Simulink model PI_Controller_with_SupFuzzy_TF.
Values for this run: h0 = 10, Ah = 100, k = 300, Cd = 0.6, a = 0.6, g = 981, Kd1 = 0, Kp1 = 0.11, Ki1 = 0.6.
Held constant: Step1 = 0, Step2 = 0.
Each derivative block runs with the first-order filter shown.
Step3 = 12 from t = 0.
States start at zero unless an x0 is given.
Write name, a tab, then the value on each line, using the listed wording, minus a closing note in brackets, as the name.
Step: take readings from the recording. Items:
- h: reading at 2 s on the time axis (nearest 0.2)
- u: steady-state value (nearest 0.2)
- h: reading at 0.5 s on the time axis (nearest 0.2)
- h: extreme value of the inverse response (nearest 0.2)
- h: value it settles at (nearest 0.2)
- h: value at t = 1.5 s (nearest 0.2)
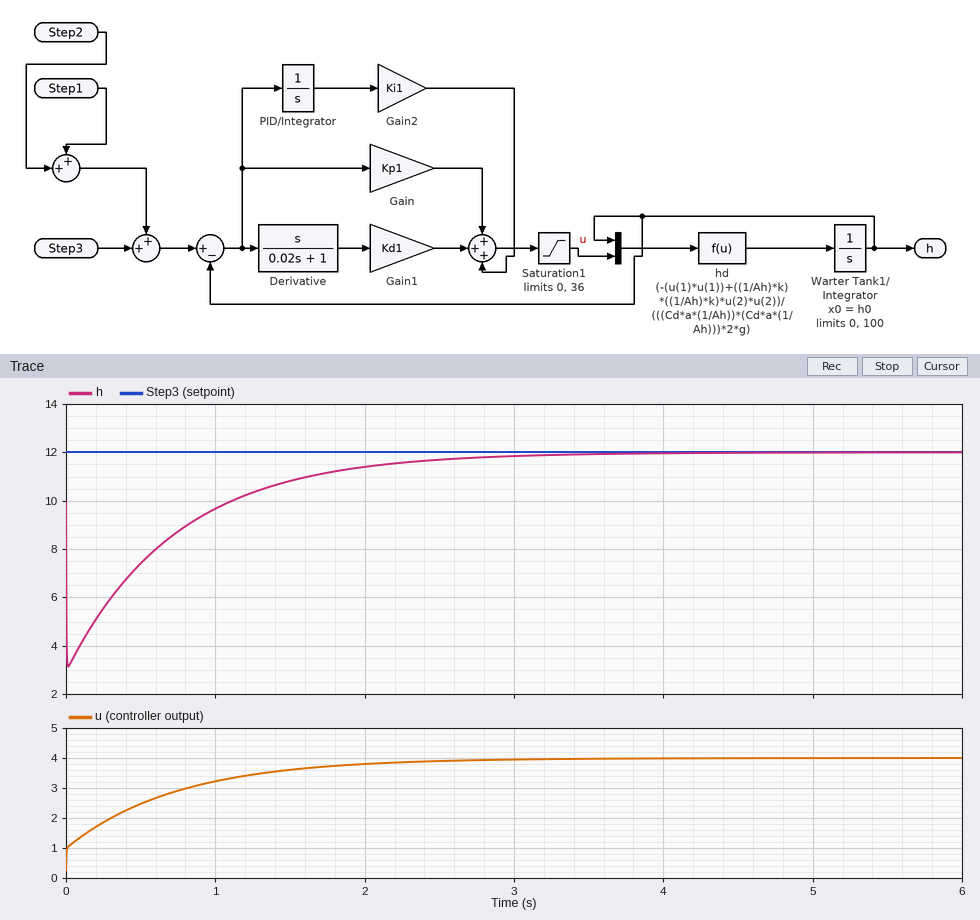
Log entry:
h: reading at 2 s on the time axis	11.4
u: steady-state value	4.0
h: reading at 0.5 s on the time axis	7.4
h: extreme value of the inverse response	3.2
h: value it settles at	12.0
h: value at t = 1.5 s	10.8
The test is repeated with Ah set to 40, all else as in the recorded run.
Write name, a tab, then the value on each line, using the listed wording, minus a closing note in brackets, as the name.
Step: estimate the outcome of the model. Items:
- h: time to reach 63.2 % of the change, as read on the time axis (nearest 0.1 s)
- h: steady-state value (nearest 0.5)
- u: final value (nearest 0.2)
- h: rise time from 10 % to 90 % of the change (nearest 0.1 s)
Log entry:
h: time to reach 63.2 % of the change, as read on the time axis	0.9 s
h: steady-state value	12.0
u: final value	1.6
h: rise time from 10 % to 90 % of the change	0.9 s
